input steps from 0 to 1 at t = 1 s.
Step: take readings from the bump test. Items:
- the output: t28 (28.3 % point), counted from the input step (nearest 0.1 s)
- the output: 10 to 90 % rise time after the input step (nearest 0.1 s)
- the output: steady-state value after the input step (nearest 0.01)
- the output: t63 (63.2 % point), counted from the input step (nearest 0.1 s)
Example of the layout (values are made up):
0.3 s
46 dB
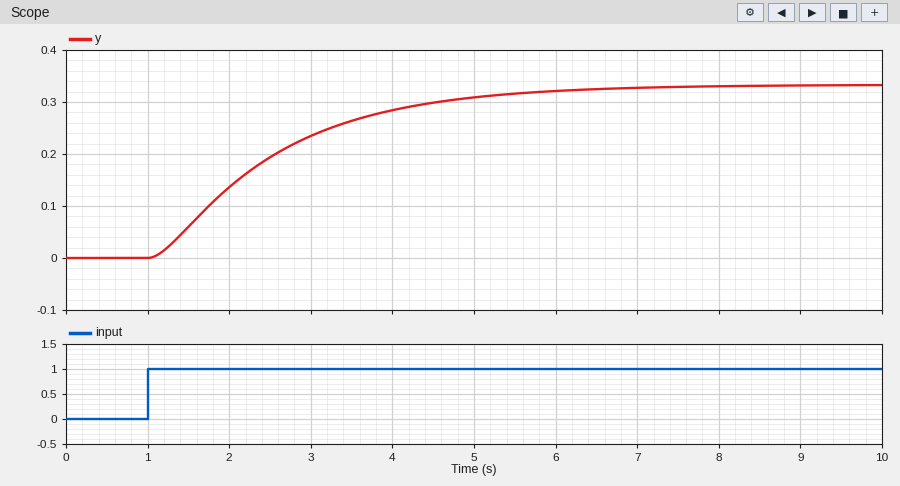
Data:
0.7 s
3.2 s
0.33
1.7 s
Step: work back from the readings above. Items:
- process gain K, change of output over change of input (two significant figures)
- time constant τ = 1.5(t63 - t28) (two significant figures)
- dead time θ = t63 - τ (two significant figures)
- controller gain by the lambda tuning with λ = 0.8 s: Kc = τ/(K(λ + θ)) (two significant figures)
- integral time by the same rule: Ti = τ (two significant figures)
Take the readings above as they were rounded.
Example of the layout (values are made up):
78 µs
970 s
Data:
0.33
1.5 s
0.20 s
4.5
1.5 s
